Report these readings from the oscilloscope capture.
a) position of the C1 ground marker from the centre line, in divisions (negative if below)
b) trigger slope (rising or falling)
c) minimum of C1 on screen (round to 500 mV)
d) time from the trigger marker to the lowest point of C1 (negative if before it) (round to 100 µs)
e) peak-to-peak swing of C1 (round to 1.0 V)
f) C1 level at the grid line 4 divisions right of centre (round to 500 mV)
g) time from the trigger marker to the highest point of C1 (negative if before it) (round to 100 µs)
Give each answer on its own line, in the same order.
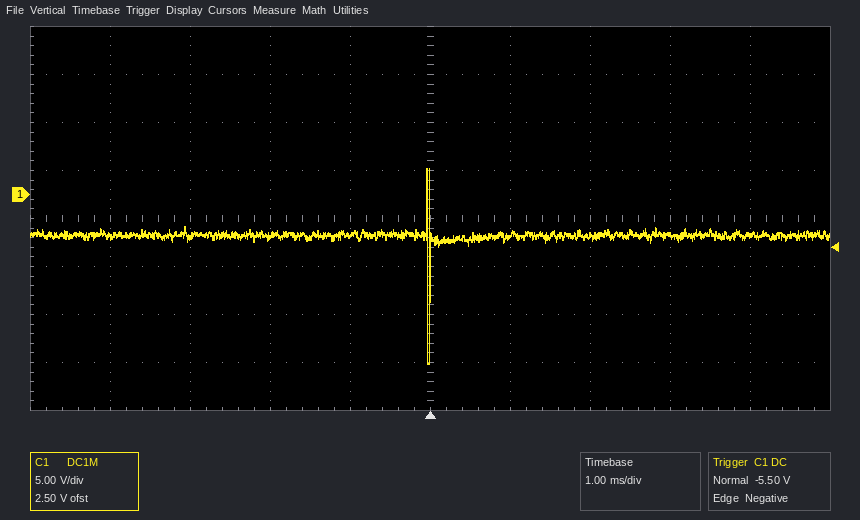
+0.5 div
falling
-17.5 V
0.0 ms
20.0 V
-4.0 V
0.0 ms
